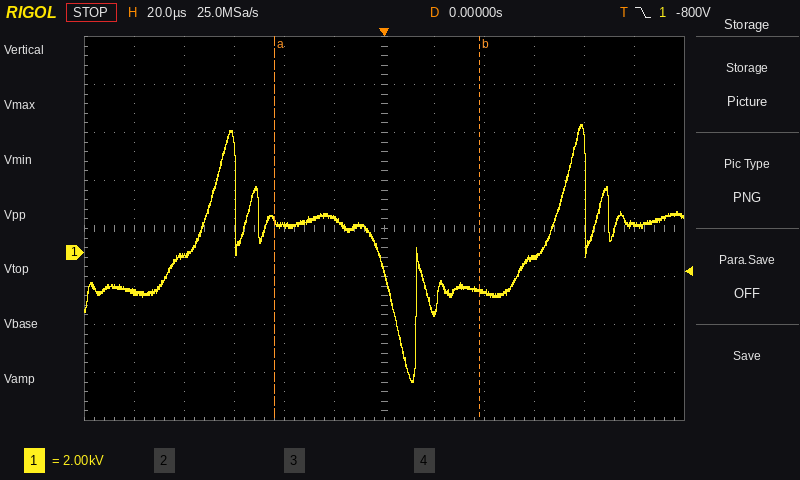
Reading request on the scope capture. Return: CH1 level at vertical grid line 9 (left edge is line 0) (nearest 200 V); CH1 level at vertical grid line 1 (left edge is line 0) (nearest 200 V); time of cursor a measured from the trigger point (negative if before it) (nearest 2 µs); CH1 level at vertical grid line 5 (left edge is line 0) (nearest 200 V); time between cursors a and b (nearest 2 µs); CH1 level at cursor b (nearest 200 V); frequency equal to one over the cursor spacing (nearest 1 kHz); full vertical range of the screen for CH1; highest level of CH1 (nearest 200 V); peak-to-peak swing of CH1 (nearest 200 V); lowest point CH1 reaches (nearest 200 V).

-200 V
-1.6 kV
-44 µs
1.4 kV
82 µs
-1.6 kV
12 kHz
16 kV
5.4 kV
10.8 kV
-5.4 kV
